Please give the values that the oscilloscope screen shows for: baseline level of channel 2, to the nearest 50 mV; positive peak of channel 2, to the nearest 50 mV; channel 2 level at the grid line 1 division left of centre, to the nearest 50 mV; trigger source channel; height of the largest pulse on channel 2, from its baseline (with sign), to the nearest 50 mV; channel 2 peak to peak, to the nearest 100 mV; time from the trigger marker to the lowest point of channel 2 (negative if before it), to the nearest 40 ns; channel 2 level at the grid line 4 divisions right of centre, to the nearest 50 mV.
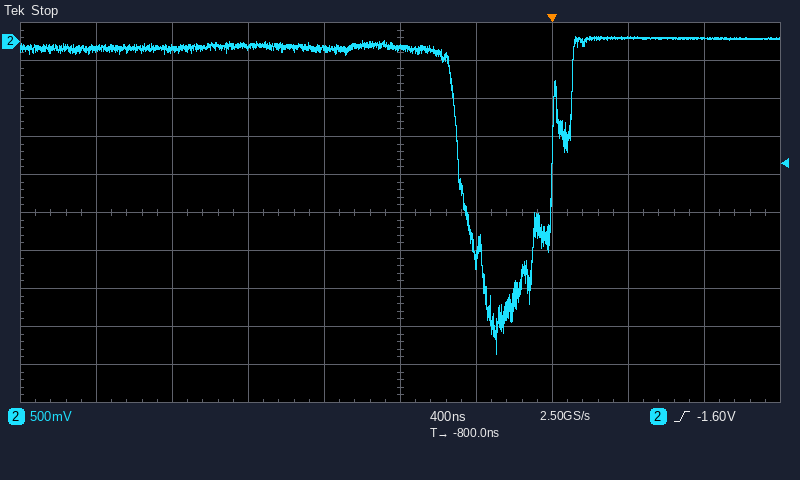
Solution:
-100 mV
50 mV
-100 mV
channel 2
-4.05 V
4.20 V
-280 ns
50 mV
